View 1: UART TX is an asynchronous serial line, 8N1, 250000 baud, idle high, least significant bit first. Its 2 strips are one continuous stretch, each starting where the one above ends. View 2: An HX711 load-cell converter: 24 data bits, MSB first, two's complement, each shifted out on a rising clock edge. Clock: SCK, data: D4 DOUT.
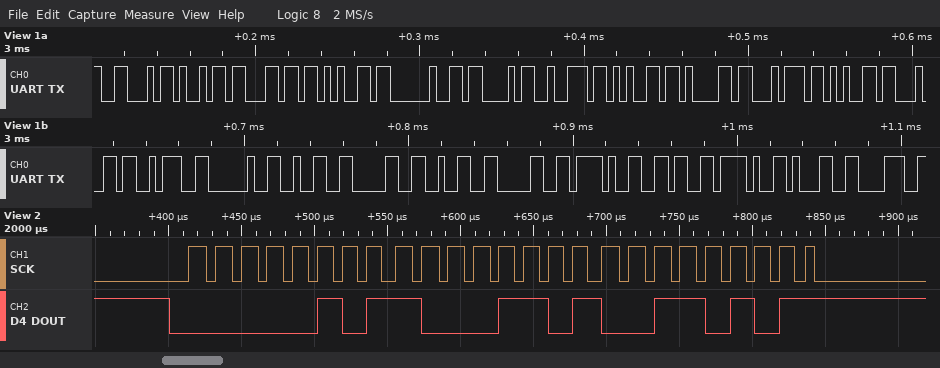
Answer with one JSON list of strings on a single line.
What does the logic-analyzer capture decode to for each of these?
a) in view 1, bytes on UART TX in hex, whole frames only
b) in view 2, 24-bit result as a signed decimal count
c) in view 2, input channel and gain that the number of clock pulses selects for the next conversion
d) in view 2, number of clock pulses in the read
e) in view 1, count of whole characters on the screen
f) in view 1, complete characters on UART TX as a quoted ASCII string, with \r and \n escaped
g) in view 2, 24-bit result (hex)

["46 69 6C 65 20 43 72 65 61 74 65 64 3A 20 32 30 32 30 2F 36 2F 31 38", "363829", "channel A, gain 128", "25", "23", "\"File Created: 2020/6/18\"", "0x058D35"]
